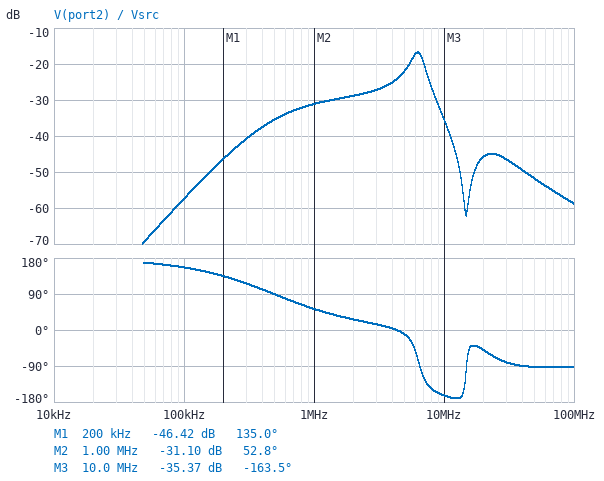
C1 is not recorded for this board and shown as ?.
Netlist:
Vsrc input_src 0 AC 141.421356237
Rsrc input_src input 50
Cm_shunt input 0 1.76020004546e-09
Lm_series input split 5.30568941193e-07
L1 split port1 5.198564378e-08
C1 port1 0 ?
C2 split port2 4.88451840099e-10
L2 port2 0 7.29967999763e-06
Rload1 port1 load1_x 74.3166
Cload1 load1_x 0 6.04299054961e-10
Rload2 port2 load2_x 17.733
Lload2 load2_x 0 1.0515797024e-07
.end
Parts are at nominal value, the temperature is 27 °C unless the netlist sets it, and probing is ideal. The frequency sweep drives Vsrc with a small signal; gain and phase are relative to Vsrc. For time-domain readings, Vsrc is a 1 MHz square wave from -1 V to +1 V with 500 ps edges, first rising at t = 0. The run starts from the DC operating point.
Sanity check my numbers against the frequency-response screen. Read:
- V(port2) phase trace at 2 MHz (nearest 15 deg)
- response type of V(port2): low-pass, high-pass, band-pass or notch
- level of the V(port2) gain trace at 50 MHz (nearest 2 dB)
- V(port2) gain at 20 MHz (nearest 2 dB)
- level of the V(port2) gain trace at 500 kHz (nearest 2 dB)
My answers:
30 deg
band-pass
-52 dB
-46 dB
-36 dB
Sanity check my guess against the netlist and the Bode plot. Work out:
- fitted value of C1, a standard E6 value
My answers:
2.2 nF
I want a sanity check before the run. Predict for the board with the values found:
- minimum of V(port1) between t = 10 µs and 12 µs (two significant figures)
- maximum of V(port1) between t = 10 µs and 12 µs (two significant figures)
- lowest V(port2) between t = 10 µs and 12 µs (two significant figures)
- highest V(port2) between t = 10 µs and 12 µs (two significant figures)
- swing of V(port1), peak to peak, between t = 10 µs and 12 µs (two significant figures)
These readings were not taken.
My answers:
-750 mV
750 mV
-93 mV
93 mV
1.5 V
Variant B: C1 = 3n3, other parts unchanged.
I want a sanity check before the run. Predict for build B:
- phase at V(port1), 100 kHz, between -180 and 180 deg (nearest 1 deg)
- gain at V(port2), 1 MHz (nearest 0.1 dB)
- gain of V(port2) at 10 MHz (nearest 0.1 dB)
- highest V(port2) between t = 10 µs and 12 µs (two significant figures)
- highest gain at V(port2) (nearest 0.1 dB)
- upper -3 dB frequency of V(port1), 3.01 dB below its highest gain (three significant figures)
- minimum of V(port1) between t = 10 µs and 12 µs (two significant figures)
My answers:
-11 deg
-32.3 dB
-43.7 dB
72 mV
-19.6 dB
528 kHz
-680 mV
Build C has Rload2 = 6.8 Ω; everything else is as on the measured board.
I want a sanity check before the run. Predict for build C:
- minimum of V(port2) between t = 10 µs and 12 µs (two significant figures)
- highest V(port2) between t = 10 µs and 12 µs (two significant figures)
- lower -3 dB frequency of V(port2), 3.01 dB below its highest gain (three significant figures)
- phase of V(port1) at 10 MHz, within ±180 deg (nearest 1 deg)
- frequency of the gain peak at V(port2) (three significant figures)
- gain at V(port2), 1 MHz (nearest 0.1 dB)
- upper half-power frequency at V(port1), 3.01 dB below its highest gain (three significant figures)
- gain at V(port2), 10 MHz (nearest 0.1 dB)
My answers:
-40 mV
40 mV
5.56 MHz
111 deg
6.30 MHz
-39.0 dB
644 kHz
-40.4 dB
